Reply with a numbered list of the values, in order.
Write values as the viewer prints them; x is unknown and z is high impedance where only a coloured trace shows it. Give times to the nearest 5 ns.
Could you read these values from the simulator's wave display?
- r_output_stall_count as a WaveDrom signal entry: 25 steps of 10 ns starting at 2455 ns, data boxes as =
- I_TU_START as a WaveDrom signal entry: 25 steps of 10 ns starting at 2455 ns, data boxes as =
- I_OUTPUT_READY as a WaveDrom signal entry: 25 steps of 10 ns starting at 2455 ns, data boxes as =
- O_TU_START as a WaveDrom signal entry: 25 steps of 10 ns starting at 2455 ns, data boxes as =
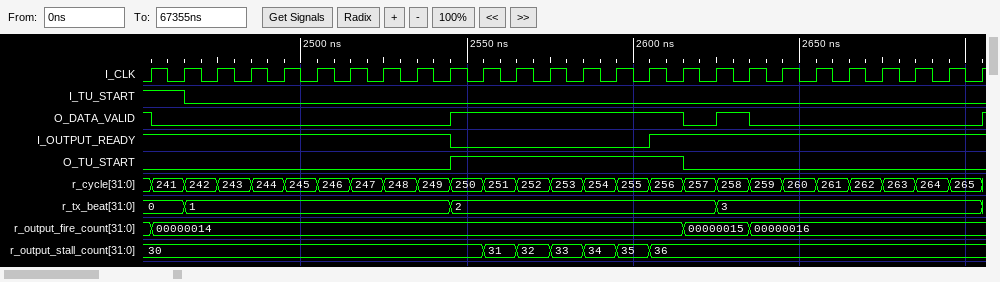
1. {name: 'r_output_stall_count', wave: '=.........======.........', data: '30 31 32 33 34 35 36'}
2. {name: 'I_TU_START', wave: '10.......................'}
3. {name: 'I_OUTPUT_READY', wave: '1........0.....1.........'}
4. {name: 'O_TU_START', wave: '0........1......0........'}
